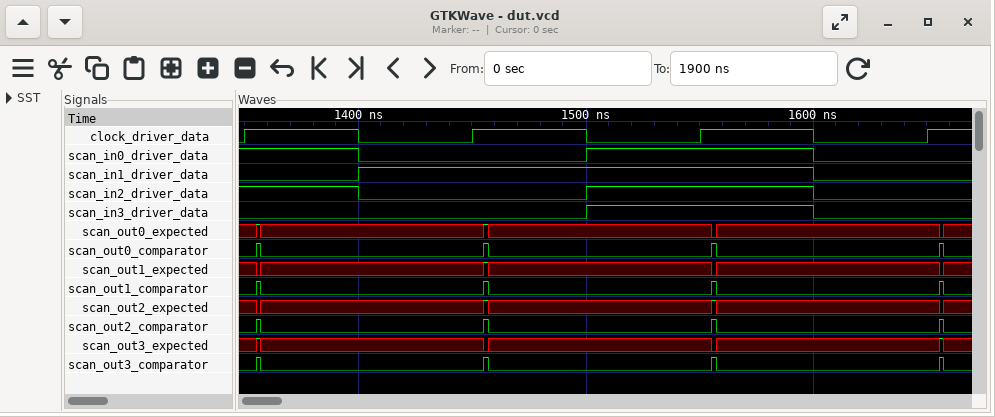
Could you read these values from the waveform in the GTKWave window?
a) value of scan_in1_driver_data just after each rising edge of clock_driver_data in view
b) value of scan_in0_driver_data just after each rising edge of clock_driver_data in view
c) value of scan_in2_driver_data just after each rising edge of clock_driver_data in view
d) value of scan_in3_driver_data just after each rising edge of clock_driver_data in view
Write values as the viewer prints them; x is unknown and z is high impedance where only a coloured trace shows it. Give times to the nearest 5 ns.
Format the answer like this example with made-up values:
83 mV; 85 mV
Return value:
0 1 1 0; 1 0 1 0; 1 0 1 0; 0 0 1 0
